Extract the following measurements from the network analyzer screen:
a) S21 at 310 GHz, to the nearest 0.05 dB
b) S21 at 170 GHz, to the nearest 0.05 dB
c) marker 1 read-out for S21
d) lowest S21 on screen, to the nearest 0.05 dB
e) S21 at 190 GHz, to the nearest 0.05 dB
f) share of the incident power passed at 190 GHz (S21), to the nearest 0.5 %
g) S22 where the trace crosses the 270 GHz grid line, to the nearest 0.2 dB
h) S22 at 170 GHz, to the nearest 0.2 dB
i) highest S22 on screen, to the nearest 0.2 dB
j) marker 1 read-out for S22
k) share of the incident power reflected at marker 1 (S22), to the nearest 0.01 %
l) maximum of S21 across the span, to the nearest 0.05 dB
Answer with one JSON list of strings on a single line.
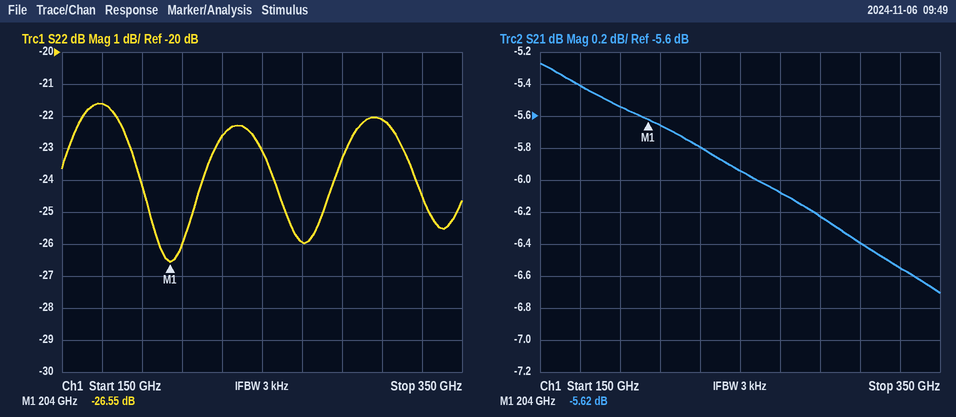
["-6.40 dB", "-5.40 dB", "-5.62 dB", "-6.70 dB", "-5.55 dB", "28.0 %", "-26.0 dB", "-21.6 dB", "-21.6 dB", "-26.55 dB", "0.22 %", "-5.25 dB"]
